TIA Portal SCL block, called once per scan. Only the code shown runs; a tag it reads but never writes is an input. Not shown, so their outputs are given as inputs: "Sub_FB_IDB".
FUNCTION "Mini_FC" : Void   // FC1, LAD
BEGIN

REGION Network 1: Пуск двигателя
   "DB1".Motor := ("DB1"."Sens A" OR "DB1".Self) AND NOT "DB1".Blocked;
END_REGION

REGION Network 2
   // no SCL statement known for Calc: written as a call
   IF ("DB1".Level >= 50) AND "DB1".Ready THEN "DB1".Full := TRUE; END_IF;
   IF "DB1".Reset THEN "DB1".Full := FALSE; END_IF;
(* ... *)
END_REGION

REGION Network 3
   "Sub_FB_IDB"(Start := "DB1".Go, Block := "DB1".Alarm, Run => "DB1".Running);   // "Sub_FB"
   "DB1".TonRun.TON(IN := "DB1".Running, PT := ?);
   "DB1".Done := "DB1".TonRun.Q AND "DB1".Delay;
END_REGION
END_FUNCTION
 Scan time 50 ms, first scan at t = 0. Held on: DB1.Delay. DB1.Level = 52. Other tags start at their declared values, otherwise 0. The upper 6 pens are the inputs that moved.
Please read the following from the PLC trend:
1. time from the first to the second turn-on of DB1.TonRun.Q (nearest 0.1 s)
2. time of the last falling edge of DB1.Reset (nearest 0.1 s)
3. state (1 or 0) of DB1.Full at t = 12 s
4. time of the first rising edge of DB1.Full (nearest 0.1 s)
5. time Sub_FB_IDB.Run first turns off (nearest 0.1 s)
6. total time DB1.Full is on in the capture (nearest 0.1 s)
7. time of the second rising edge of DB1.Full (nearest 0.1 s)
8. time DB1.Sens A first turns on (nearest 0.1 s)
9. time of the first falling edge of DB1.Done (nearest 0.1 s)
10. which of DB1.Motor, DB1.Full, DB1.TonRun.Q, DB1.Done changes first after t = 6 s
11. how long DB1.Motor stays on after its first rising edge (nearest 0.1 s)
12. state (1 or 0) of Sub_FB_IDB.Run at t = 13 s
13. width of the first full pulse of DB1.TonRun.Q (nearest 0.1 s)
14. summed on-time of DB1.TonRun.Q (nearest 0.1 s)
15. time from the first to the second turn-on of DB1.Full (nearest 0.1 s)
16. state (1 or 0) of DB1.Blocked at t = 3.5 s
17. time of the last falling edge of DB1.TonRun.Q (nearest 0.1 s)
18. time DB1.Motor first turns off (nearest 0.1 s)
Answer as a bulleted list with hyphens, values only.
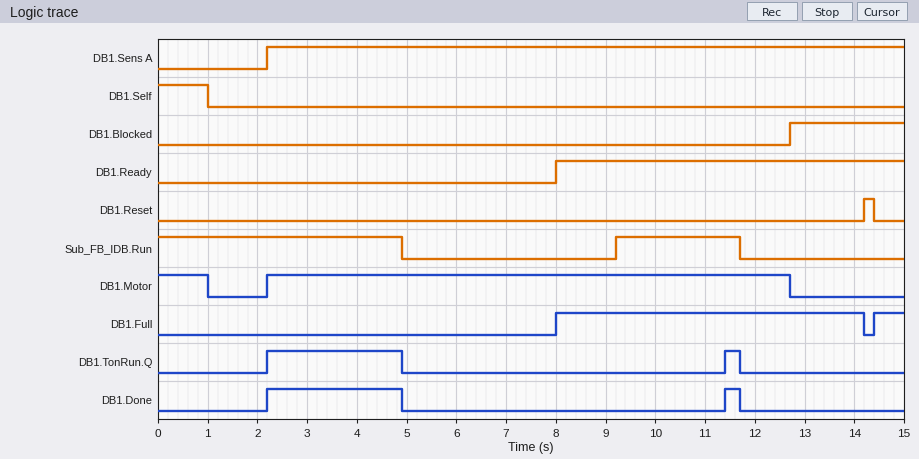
- 9.2 s
- 14.4 s
- 1
- 8.0 s
- 4.9 s
- 6.8 s
- 14.4 s
- 2.2 s
- 4.9 s
- DB1.Full
- 10.5 s
- 0
- 2.7 s
- 3.0 s
- 6.4 s
- 0
- 11.7 s
- 1.0 s
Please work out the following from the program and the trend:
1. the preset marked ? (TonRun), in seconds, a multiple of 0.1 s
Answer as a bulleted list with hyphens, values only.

- 2.2 s
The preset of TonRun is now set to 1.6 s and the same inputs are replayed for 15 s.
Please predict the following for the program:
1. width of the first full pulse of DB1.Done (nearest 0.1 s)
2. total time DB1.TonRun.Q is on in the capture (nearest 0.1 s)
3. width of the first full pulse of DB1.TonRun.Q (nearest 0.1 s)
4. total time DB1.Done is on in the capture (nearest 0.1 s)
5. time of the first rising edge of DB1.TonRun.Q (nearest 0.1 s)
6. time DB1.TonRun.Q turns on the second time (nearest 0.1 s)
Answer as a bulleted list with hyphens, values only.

- 3.3 s
- 4.2 s
- 3.3 s
- 4.2 s
- 1.6 s
- 10.8 s
